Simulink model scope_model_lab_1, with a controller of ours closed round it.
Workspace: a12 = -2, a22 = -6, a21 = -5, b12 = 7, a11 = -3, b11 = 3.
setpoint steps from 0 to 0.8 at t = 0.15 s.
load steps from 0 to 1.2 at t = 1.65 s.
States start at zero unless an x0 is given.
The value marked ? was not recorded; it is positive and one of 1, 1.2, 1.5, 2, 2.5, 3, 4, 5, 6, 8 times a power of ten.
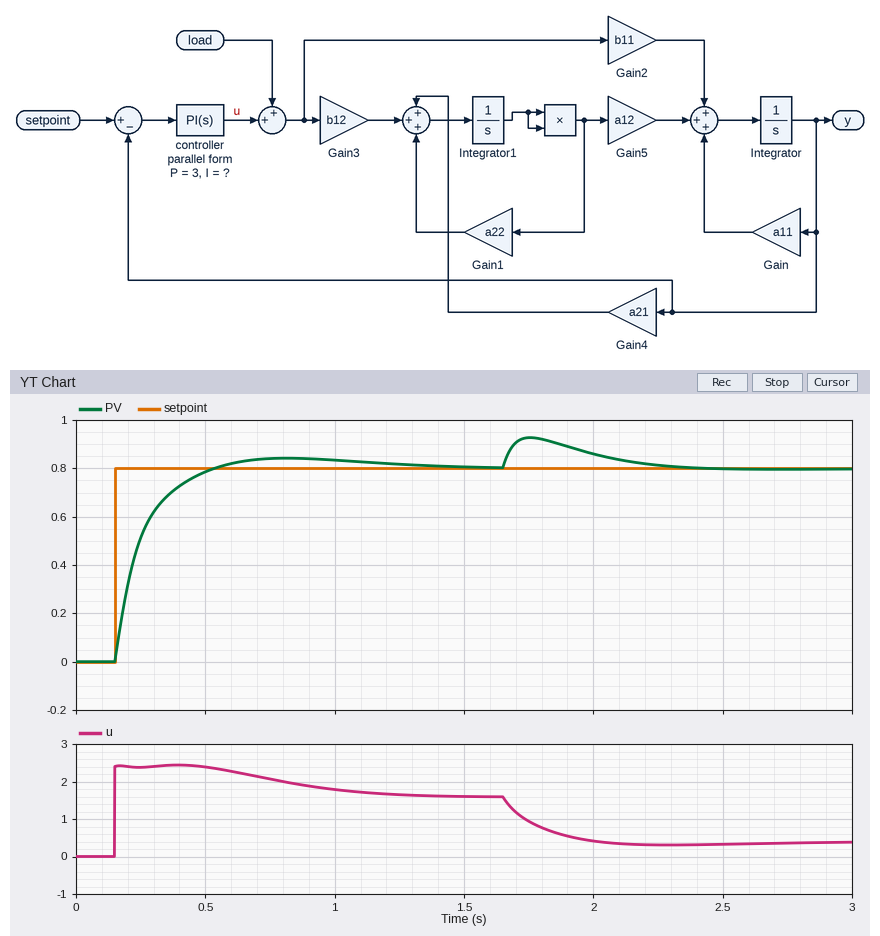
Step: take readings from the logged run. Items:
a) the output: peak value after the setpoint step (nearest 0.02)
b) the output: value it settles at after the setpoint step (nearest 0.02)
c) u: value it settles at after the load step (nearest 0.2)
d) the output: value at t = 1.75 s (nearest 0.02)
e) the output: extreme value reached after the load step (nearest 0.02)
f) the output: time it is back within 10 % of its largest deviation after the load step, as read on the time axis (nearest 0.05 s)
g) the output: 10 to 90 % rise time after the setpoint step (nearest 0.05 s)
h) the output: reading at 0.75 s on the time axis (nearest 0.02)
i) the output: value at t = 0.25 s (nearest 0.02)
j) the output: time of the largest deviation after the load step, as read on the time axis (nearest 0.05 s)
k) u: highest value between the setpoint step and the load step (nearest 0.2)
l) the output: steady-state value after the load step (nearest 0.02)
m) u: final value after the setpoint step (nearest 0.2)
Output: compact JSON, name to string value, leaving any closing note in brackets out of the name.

{"the output: peak value after the setpoint step": "0.84", "the output: value it settles at after the setpoint step": "0.80", "u: value it settles at after the load step": "0.4", "the output: value at t = 1.75 s": "0.92", "the output: extreme value reached after the load step": "0.92", "the output: time it is back within 10 % of its largest deviation after the load step, as read on the time axis": "2.25 s", "the output: 10 to 90 % rise time after the setpoint step": "0.25 s", "the output: reading at 0.75 s on the time axis": "0.84", "the output: value at t = 0.25 s": "0.52", "the output: time of the largest deviation after the load step, as read on the time axis": "1.75 s", "u: highest value between the setpoint step and the load step": "2.4", "the output: steady-state value after the load step": "0.80", "u: final value after the setpoint step": "1.6"}
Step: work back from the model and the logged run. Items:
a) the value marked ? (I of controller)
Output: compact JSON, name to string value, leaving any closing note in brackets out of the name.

{"the value marked ?": "30"}
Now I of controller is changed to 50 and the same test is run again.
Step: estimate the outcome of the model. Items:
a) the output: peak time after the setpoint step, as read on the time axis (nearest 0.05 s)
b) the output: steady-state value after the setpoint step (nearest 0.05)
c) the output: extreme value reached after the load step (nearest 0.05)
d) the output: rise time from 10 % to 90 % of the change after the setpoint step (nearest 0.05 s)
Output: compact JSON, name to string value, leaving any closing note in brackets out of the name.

{"the output: peak time after the setpoint step, as read on the time axis": "0.55 s", "the output: steady-state value after the setpoint step": "0.80", "the output: extreme value reached after the load step": "0.90", "the output: rise time from 10 % to 90 % of the change after the setpoint step": "0.15 s"}
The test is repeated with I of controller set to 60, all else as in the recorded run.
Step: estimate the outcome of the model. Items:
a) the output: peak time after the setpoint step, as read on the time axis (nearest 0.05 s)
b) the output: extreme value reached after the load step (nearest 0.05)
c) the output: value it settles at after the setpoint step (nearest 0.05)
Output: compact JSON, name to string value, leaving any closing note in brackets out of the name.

{"the output: peak time after the setpoint step, as read on the time axis": "0.50 s", "the output: extreme value reached after the load step": "0.90", "the output: value it settles at after the setpoint step": "0.80"}
